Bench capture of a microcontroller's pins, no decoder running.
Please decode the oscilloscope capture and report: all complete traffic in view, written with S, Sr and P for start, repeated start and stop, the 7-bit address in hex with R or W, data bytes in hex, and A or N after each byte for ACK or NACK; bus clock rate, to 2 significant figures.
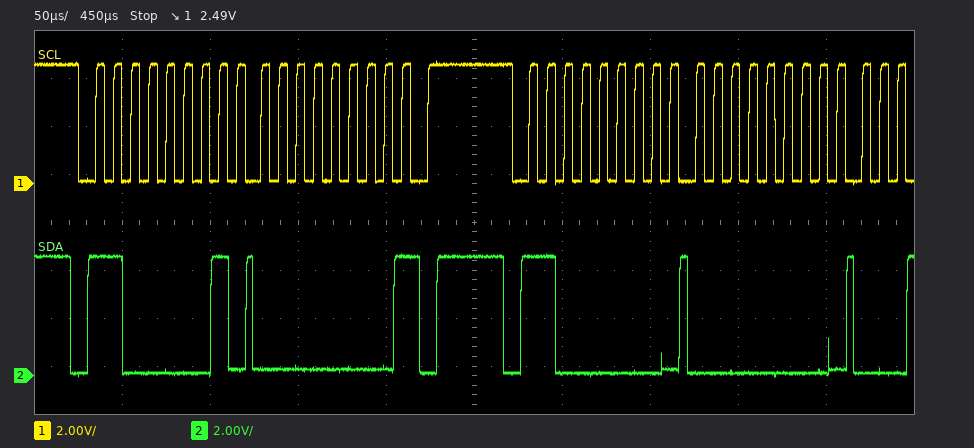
S 60R A 00 N P S 60W A 00 A
100 kHz
